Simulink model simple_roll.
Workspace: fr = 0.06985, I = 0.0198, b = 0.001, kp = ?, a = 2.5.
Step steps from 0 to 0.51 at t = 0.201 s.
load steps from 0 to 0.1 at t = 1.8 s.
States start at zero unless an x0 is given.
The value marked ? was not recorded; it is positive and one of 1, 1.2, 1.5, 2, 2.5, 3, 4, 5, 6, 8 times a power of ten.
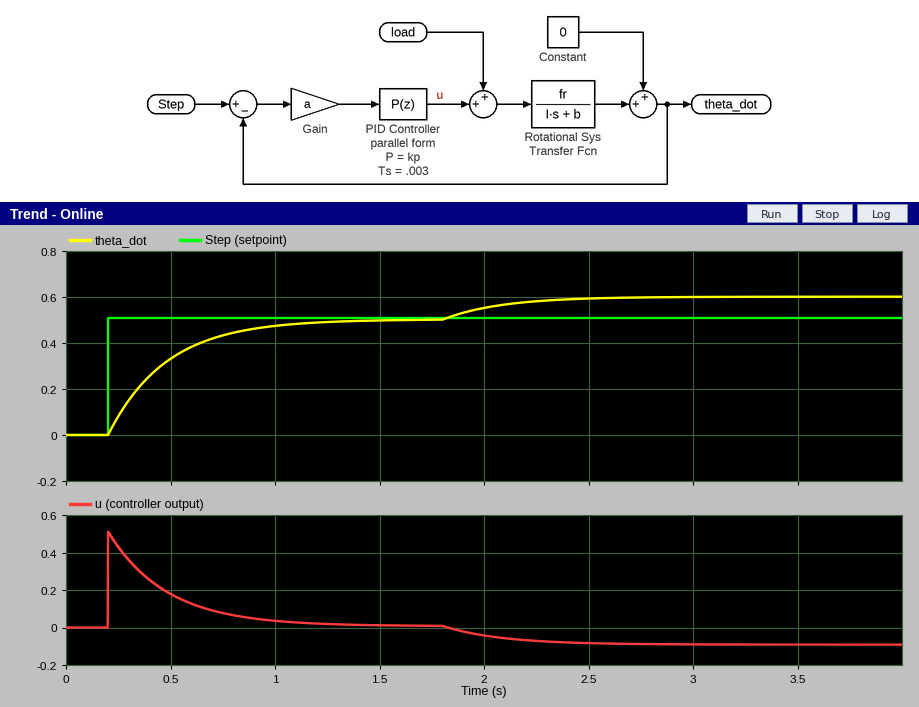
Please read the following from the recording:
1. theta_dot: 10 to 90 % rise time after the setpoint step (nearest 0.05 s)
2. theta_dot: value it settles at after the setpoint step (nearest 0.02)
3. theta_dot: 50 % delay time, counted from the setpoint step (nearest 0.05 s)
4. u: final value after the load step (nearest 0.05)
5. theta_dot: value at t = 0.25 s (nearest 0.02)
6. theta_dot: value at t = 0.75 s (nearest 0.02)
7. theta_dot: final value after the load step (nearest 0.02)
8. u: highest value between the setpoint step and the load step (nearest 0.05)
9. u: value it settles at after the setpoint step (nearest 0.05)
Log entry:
0.60 s
0.50
0.20 s
-0.10
0.08
0.44
0.60
0.50
0.00
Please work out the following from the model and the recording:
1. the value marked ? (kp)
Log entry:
0.4
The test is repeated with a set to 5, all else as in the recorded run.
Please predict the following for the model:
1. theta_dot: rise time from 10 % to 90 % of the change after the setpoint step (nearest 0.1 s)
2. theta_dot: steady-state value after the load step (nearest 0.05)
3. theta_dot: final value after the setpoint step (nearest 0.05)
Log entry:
0.3 s
0.55
0.50
